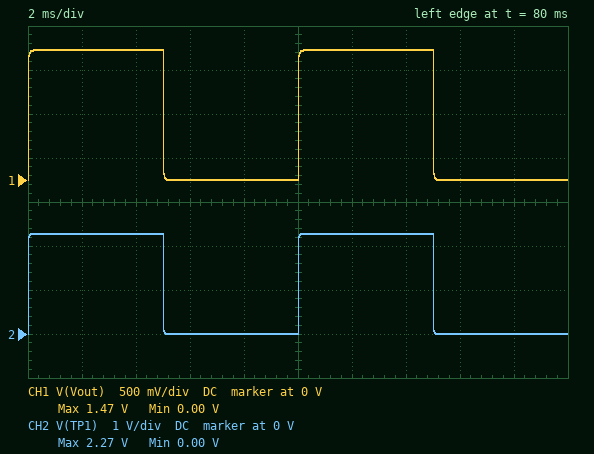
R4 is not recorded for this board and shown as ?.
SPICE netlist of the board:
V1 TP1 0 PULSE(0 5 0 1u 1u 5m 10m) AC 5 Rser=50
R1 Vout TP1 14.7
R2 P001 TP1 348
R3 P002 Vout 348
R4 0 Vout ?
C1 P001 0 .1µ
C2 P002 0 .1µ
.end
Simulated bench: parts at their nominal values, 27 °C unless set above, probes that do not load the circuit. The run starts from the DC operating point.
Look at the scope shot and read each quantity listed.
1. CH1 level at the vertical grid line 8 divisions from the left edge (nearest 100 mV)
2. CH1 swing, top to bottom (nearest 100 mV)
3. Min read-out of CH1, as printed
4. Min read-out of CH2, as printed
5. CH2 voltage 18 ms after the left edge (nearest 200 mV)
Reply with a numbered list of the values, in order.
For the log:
1. 0 V
2. 1.5 V
3. 0.00 V
4. 0.00 V
5. 0 V
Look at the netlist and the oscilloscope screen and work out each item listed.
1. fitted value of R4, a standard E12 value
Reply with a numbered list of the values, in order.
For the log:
1. 27 Ω
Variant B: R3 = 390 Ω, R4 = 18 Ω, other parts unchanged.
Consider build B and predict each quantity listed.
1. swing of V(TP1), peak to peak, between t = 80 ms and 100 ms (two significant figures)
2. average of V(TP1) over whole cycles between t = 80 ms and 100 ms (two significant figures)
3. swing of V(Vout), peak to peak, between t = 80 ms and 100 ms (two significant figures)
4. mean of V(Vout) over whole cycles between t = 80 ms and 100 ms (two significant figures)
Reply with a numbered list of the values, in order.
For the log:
1. 2.0 V
2. 990 mV
3. 1.1 V
4. 540 mV
